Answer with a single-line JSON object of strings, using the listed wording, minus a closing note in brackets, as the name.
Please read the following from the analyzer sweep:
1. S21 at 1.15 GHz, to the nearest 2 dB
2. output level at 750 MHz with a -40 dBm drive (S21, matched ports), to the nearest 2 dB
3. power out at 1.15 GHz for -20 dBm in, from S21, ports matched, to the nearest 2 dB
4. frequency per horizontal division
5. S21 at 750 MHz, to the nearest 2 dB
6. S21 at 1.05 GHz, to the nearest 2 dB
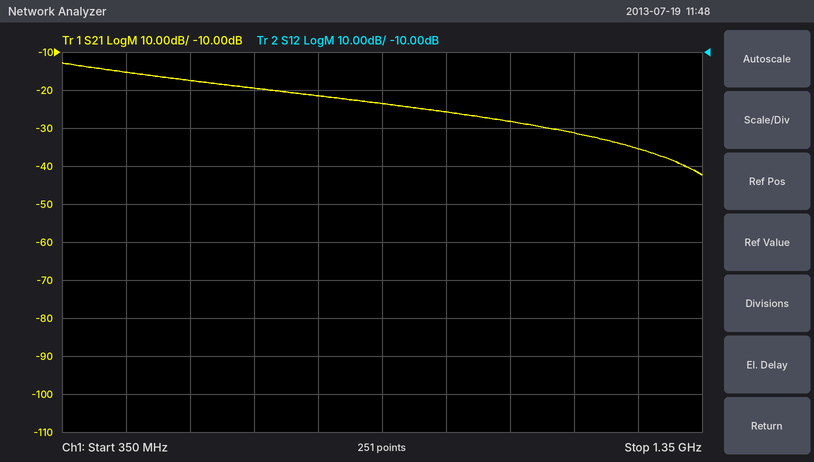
{"S21 at 1.15 GHz, to the nearest 2 dB": "-32 dB", "output level at 750 MHz with a -40 dBm drive (S21, matched ports), to the nearest 2 dB": "-62 dBm", "power out at 1.15 GHz for -20 dBm in, from S21, ports matched, to the nearest 2 dB": "-52 dBm", "frequency per horizontal division": "100 MHz", "S21 at 750 MHz, to the nearest 2 dB": "-22 dB", "S21 at 1.05 GHz, to the nearest 2 dB": "-28 dB"}
